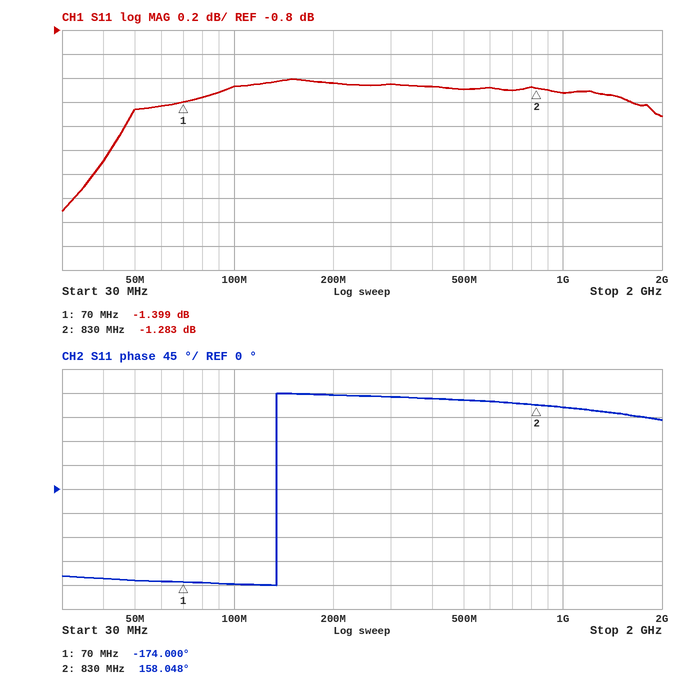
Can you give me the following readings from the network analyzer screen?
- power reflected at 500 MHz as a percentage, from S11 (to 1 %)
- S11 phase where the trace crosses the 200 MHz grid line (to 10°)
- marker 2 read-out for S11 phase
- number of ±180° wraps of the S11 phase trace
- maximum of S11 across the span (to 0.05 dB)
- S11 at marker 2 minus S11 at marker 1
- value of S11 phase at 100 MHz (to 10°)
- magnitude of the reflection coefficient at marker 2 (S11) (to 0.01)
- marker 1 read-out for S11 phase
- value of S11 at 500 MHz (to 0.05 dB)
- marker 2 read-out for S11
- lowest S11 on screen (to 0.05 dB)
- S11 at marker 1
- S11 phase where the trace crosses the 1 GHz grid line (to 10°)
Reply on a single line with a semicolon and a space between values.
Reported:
74 %; 180°; 158.048°; 1; -1.20 dB; 0.116 dB; -180°; 0.86; -174.000°; -1.30 dB; -1.283 dB; -2.30 dB; -1.399 dB; 150°
